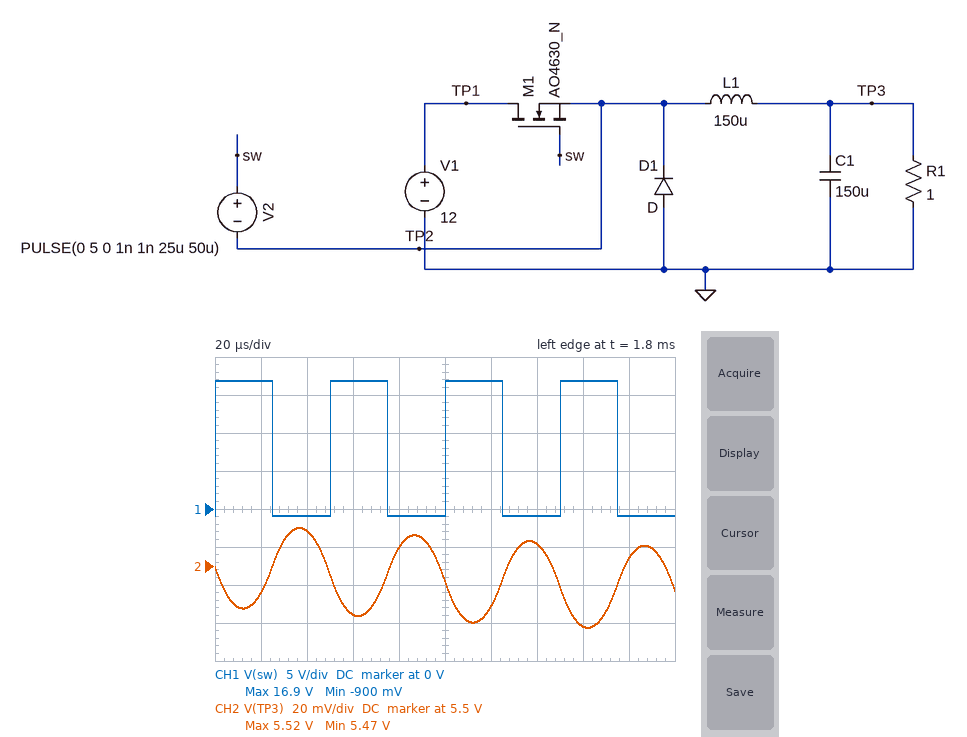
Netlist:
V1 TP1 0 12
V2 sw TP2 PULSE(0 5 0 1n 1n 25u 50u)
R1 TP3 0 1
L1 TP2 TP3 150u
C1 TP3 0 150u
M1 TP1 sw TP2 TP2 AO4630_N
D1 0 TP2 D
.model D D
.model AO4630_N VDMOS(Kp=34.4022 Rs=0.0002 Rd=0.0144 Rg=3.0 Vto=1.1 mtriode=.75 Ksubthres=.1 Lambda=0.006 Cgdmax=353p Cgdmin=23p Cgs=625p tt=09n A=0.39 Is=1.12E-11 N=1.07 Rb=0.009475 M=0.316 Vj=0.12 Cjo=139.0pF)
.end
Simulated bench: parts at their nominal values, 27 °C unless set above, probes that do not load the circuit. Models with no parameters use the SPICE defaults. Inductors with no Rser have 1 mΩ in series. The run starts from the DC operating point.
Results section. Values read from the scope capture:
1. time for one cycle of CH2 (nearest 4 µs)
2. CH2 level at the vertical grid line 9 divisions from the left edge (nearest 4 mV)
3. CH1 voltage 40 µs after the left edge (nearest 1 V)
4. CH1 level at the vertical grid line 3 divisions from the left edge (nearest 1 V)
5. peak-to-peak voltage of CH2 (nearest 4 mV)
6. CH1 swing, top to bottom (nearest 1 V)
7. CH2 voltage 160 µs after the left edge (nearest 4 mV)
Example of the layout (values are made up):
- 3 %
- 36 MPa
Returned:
- 52 µs
- 5.504 V
- -1 V
- 17 V
- 52 mV
- 18 V
- 5.468 V
